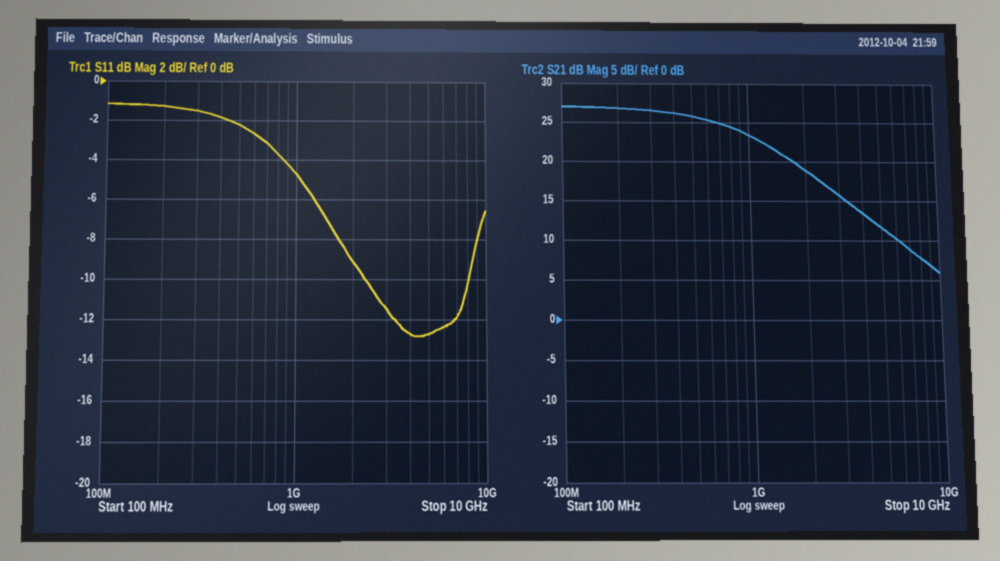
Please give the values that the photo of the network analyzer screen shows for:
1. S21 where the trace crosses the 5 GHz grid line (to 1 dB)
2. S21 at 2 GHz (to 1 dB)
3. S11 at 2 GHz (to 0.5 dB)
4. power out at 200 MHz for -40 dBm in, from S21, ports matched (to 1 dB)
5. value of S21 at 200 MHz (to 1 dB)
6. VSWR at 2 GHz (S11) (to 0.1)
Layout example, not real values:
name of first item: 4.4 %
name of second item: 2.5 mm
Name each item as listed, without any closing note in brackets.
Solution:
S21 where the trace crosses the 5 GHz grid line: 12 dB
S21 at 2 GHz: 19 dB
S11 at 2 GHz: -9.0 dB
power out at 200 MHz for -40 dBm in, from S21, ports matched: -13 dBm
value of S21 at 200 MHz: 27 dB
VSWR at 2 GHz (S11): 2.1
